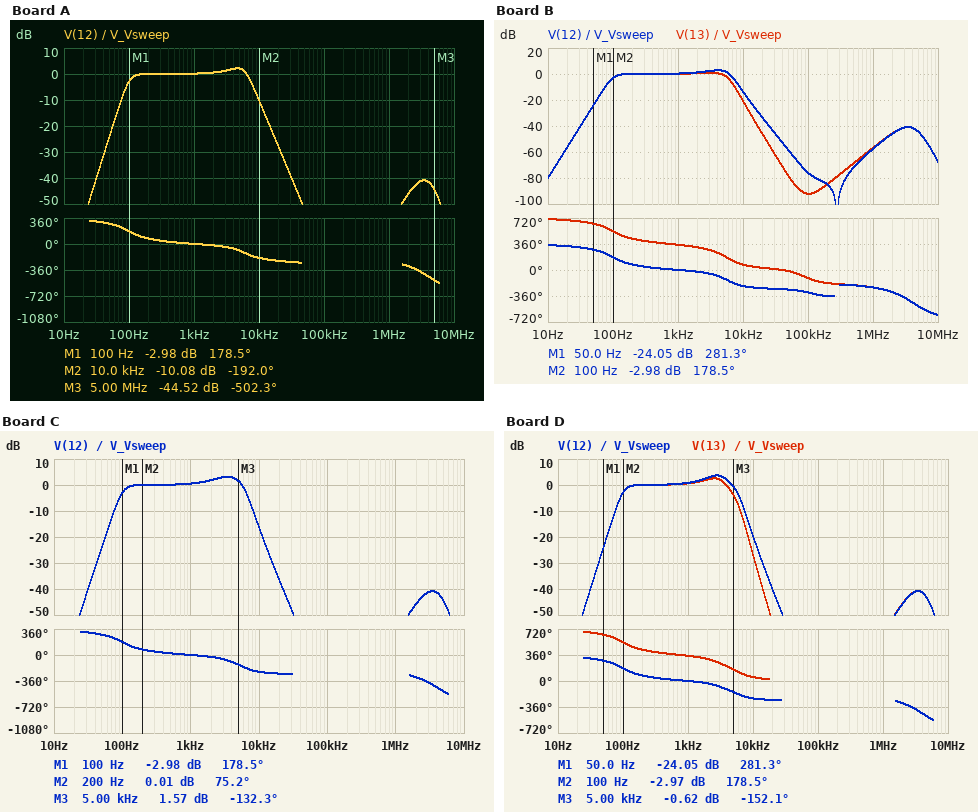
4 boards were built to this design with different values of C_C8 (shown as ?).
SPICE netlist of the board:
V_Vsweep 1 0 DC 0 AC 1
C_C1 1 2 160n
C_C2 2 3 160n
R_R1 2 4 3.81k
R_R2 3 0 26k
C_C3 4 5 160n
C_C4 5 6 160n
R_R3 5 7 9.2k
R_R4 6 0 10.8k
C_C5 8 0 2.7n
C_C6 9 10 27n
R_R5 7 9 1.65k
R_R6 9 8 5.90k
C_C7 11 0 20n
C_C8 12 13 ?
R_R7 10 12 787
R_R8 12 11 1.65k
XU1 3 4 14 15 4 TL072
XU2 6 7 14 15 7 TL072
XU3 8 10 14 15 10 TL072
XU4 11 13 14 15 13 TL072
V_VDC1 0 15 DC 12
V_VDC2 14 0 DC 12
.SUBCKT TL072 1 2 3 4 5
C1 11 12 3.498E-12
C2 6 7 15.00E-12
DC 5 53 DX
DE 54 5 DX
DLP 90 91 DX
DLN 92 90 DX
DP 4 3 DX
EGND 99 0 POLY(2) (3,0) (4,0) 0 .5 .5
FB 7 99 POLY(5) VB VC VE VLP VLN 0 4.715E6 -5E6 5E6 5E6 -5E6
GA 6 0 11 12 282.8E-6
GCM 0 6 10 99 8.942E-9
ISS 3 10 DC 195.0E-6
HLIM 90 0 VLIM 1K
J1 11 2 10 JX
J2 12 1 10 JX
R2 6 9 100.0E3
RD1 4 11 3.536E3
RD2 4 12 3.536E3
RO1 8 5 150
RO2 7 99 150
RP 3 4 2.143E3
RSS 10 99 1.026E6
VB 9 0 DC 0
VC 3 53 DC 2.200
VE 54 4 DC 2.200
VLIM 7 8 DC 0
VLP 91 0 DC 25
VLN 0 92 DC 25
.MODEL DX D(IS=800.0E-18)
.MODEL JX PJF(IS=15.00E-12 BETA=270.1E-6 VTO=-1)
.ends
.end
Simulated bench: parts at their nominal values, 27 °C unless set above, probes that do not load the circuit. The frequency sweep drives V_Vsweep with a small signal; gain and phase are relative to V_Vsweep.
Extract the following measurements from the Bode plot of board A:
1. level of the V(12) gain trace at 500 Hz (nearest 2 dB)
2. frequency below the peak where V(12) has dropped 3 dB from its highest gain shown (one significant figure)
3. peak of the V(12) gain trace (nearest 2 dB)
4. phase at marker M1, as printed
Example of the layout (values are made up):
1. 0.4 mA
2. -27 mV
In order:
1. 0 dB
2. 100 Hz
3. 2 dB
4. 178.5 deg
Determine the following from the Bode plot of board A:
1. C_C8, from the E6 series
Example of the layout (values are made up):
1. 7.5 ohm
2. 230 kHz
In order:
1. 22 nF
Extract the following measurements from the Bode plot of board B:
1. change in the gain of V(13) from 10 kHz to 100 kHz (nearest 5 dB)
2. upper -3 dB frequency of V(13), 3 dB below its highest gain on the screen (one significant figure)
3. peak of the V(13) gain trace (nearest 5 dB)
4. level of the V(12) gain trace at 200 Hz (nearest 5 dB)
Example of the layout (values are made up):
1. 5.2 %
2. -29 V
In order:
1. -70 dB
2. 6 kHz
3. 0 dB
4. 0 dB
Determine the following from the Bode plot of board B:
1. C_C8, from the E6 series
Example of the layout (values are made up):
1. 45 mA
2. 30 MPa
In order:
1. 47 nF
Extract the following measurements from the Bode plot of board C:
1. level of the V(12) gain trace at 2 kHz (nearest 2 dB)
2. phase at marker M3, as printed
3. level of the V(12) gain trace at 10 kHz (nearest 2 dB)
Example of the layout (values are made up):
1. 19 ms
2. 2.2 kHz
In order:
1. 2 dB
2. -132.3 deg
3. -16 dB
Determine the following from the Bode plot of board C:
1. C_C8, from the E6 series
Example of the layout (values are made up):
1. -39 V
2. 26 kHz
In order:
1. 68 nF
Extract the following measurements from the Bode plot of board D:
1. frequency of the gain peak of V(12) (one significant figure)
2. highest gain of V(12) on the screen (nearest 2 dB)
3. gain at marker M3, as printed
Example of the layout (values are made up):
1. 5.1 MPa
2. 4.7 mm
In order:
1. 3 kHz
2. 4 dB
3. -0.62 dB
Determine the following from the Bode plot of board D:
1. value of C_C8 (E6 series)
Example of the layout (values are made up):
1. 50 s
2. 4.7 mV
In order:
1. 100 nF
